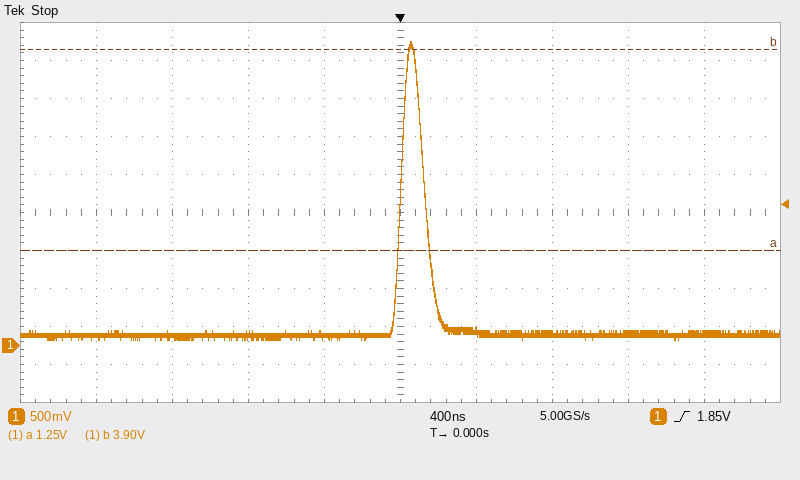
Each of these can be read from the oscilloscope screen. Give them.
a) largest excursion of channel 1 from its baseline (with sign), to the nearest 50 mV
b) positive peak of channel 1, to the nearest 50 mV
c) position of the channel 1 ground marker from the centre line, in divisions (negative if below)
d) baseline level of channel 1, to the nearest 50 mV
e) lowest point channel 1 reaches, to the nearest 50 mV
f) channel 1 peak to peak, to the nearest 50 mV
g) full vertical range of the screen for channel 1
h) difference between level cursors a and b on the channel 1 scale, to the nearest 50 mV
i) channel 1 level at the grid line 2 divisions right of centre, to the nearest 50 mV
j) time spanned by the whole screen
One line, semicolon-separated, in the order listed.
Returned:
+3.85 V; 4.00 V; -3.5 div; 150 mV; 100 mV; 3.90 V; 5 V; 2.65 V; 150 mV; 4 µs
